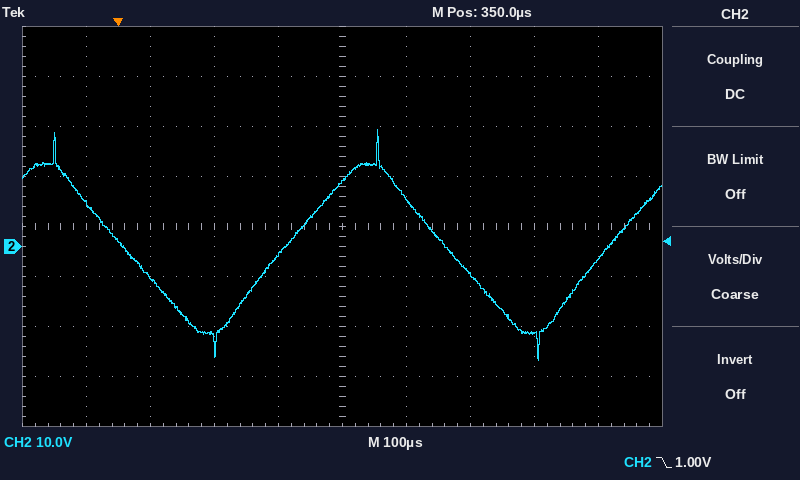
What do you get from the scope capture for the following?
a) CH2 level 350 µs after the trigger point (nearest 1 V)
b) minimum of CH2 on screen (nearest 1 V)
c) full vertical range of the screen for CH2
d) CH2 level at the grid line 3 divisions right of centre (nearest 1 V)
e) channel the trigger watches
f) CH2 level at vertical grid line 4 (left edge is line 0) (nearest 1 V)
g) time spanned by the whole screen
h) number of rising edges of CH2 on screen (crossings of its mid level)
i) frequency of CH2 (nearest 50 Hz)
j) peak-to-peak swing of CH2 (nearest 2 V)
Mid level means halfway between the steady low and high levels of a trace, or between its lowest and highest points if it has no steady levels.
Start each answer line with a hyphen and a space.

- 13 V
- -23 V
- 80 V
- -18 V
- CH2
- -2 V
- 1 ms
- 2
- 2.00 kHz
- 46 V
